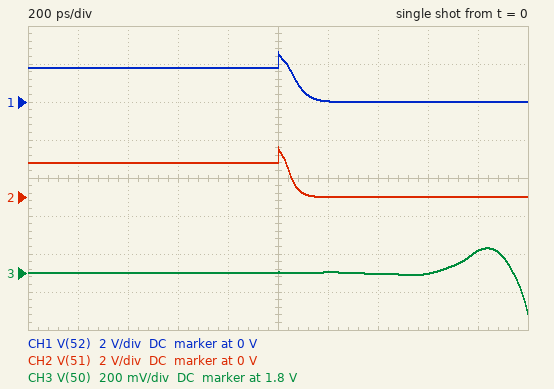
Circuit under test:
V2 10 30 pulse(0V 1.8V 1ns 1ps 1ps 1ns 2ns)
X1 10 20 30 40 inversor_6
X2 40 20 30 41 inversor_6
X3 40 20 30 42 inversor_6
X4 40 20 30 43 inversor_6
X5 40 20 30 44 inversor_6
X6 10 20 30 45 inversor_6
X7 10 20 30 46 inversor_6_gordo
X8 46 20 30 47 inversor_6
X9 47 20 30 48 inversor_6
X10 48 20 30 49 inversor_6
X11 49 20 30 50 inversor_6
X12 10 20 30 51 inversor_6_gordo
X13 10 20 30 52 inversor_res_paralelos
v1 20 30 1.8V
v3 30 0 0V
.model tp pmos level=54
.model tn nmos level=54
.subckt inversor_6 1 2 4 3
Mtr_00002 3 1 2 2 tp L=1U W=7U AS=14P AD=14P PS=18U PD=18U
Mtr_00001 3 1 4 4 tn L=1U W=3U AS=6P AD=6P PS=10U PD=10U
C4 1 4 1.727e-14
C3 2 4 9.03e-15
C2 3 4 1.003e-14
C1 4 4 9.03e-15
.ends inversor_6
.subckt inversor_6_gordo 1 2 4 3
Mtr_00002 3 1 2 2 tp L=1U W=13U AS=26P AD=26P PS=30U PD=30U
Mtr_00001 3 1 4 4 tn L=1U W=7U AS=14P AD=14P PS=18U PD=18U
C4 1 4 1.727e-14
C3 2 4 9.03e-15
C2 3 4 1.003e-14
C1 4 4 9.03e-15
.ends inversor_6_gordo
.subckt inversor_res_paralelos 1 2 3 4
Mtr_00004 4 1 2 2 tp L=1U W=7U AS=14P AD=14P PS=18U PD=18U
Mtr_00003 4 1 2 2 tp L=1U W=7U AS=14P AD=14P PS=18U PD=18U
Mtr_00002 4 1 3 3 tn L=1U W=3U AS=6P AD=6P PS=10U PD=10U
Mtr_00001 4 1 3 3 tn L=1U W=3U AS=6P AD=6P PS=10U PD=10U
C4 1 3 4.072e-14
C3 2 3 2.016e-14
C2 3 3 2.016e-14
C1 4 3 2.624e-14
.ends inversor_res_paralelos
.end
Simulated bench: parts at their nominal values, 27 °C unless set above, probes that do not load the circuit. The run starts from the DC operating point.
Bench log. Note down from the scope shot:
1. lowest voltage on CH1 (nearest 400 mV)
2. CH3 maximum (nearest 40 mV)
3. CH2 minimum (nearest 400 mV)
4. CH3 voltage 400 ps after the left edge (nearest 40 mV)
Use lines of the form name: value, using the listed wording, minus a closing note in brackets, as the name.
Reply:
lowest voltage on CH1: 0 V
CH3 maximum: 1.92 V
CH2 minimum: 0 V
CH3 voltage 400 ps after the left edge: 1.80 V
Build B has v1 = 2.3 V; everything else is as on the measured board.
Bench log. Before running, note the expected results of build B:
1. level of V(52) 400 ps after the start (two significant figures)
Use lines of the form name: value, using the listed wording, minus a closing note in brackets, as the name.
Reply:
level of V(52) 400 ps after the start: 2.3 V
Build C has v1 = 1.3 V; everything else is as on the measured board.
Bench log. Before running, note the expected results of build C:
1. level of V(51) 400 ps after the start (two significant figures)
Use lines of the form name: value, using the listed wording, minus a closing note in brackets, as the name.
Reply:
level of V(51) 400 ps after the start: 1.3 V
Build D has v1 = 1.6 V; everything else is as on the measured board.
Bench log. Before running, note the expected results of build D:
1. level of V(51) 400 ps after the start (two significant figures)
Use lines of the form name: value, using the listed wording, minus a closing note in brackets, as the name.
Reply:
level of V(51) 400 ps after the start: 1.6 V
